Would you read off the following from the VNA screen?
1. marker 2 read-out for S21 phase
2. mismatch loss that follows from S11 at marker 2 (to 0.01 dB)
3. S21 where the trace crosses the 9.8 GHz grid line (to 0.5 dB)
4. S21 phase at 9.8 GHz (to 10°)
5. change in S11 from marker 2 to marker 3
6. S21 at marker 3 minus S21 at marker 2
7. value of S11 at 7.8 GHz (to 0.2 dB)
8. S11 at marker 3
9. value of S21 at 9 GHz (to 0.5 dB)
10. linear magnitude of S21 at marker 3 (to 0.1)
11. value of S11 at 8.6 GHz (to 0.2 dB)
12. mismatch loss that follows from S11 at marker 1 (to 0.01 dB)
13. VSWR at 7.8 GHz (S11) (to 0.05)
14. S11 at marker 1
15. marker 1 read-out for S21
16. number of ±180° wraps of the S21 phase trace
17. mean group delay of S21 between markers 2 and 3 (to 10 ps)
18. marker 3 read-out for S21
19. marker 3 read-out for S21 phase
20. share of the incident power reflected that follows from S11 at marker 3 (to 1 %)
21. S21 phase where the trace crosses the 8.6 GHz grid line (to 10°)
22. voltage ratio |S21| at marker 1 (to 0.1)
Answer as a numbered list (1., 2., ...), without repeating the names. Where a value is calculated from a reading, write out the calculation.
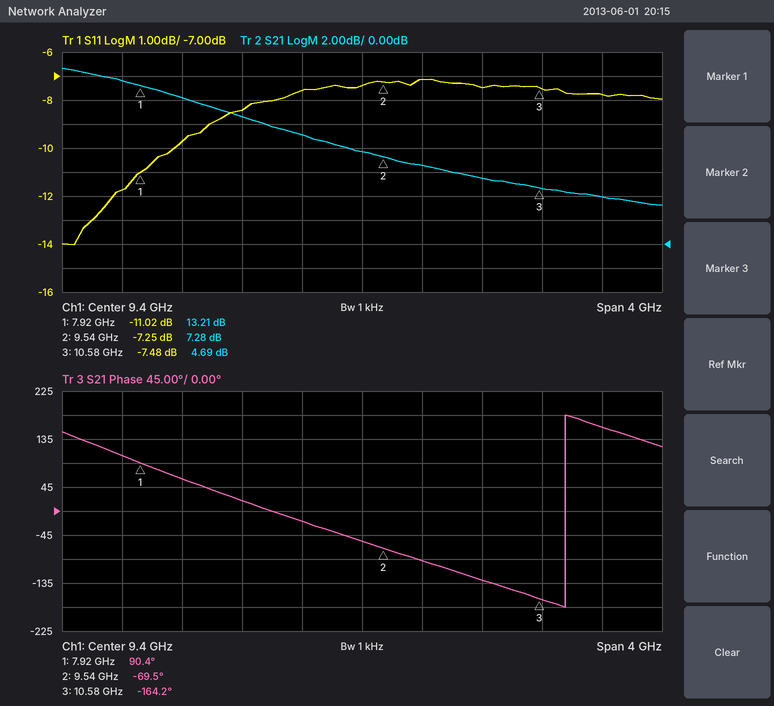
1. -69.5°
2. −10 log10(1 − 10^(-7.25/10)) ≈ 0.91 dB
3. 6.5 dB
4. -90°
5. -7.48 − (-7.25) = -0.23 dB
6. 4.69 − (7.28) = -2.59 dB
7. -11.8 dB
8. -7.48 dB
9. 9.0 dB
10. 10^(4.69/20) ≈ 1.7
11. -8.4 dB
12. −10 log10(1 − 10^(-11.02/10)) ≈ 0.36 dB
13. |Γ| = 10^(-11.8/20) = 0.2570; VSWR = (1 + 0.2570)/(1 − 0.2570) ≈ 1.69, so 1.70 to the nearest 0.05
14. -11.02 dB
15. 13.21 dB
16. 1
17. −(-164.2° − (-69.5°))/(360° × 1.04 GHz) ≈ 253 ps, so 250 ps to the nearest 10 ps
18. 4.69 dB
19. -164.2°
20. 10^(-7.48/10) ≈ 18 %
21. 20°
22. 10^(13.21/20) ≈ 4.6
